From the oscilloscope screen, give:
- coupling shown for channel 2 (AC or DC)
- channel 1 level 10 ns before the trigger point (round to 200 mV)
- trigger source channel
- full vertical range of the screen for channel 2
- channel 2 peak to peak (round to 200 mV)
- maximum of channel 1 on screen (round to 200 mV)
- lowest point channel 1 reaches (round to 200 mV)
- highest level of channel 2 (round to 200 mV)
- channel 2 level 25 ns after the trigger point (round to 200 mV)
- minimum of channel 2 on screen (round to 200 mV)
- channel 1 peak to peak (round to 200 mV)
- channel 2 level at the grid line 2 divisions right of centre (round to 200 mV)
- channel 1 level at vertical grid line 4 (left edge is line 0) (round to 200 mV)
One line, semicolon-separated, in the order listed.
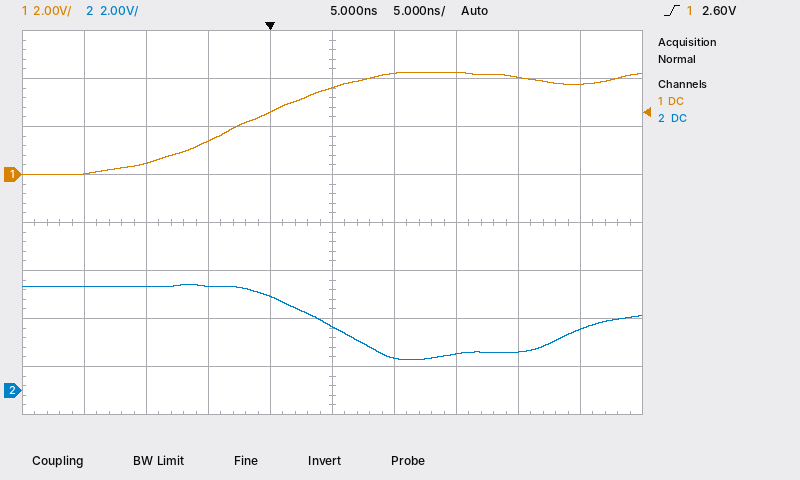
DC; 400 mV; channel 1; 16 V; 3.2 V; 4.2 V; 0.0 V; 4.4 V; 2.6 V; 1.2 V; 4.2 V; 1.6 V; 2.6 V
